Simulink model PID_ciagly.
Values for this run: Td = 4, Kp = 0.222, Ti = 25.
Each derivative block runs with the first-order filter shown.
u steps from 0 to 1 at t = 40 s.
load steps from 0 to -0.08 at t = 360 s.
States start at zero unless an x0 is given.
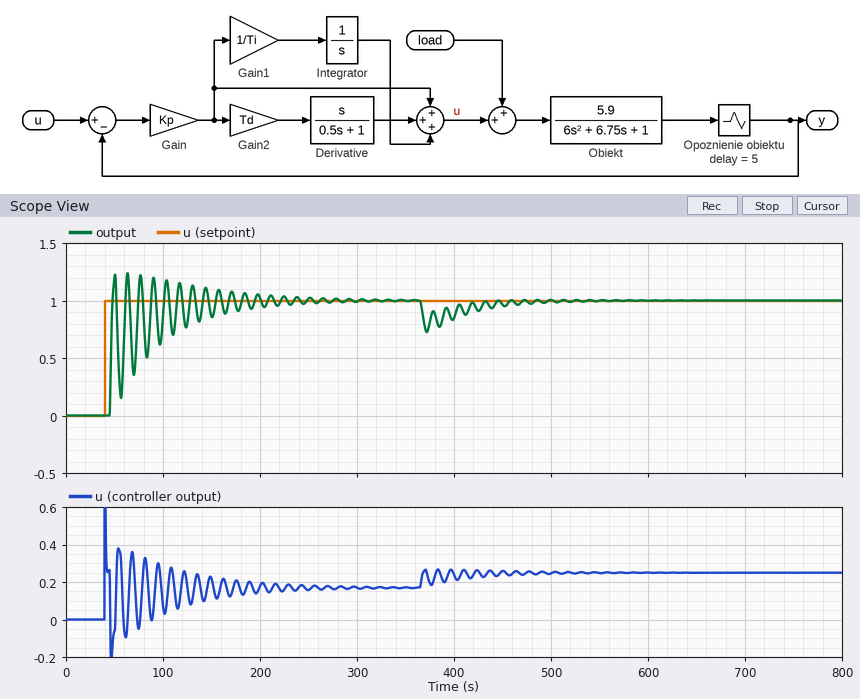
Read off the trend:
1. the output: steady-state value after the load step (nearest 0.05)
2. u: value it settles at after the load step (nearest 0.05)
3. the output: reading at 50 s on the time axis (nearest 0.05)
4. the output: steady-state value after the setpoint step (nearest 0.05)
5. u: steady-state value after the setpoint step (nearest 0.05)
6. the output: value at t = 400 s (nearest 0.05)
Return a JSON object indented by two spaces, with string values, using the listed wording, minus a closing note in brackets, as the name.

{
  "the output: steady-state value after the load step": "1.00",
  "u: value it settles at after the load step": "0.25",
  "the output: reading at 50 s on the time axis": "1.20",
  "the output: steady-state value after the setpoint step": "1.00",
  "u: steady-state value after the setpoint step": "0.15",
  "the output: value at t = 400 s": "0.85"
}
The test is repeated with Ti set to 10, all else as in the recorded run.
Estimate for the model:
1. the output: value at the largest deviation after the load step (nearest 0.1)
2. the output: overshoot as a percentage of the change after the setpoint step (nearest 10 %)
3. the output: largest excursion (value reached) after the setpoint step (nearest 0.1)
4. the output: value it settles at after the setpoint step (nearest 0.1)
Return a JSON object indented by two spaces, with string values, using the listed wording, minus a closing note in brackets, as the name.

{
  "the output: value at the largest deviation after the load step": "0.7",
  "the output: overshoot as a percentage of the change after the setpoint step": "40 %",
  "the output: largest excursion (value reached) after the setpoint step": "1.4",
  "the output: value it settles at after the setpoint step": "1.0"
}
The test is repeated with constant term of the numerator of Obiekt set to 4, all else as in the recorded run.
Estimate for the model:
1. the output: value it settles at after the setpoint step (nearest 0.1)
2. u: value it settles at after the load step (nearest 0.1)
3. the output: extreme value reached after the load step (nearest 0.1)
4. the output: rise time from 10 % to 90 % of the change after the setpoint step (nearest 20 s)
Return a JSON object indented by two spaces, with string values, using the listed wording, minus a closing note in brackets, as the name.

{
  "the output: value it settles at after the setpoint step": "1.0",
  "u: value it settles at after the load step": "0.3",
  "the output: extreme value reached after the load step": "0.8",
  "the output: rise time from 10 % to 90 % of the change after the setpoint step": "80 s"
}
